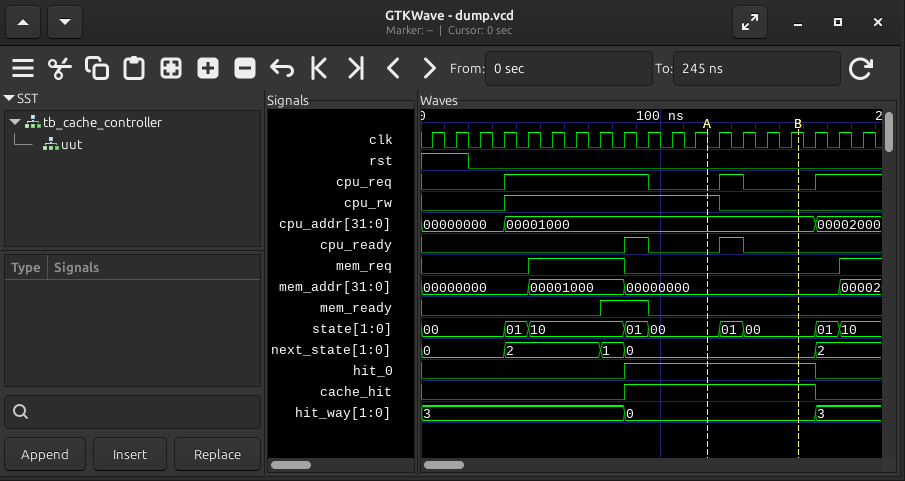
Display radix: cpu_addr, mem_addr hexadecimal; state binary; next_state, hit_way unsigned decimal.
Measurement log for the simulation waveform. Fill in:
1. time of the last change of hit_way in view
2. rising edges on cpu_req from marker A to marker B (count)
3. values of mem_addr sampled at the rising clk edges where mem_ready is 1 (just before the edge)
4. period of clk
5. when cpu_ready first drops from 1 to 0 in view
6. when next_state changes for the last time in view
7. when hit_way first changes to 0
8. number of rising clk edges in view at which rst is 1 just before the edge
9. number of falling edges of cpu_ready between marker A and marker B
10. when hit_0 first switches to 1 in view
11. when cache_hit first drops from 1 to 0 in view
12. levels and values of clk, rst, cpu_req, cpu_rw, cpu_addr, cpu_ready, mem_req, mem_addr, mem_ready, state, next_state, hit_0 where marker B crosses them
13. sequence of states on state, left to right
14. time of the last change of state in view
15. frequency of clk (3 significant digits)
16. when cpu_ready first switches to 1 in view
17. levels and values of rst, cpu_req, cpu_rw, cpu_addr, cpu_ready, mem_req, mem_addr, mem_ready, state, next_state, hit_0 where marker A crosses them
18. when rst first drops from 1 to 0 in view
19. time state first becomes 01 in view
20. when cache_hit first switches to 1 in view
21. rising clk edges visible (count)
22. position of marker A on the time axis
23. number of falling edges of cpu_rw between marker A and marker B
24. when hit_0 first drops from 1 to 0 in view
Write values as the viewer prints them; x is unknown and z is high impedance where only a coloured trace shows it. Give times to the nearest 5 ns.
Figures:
165 ns
1
00001000, 00000000
10 ns
95 ns
165 ns
85 ns
2
1
85 ns
165 ns
clk=1, rst=0, cpu_req=0, cpu_rw=0, cpu_addr=00001000, cpu_ready=0, mem_req=0, mem_addr=00000000, mem_ready=0, state=00, next_state=0, hit_0=1
00, 01, 10, 01, 00, 01, 00, 01, 10
175 ns
100 MHz
85 ns
rst=0, cpu_req=0, cpu_rw=1, cpu_addr=00001000, cpu_ready=0, mem_req=0, mem_addr=00000000, mem_ready=0, state=00, next_state=0, hit_0=1
20 ns
35 ns
85 ns
19
120 ns
1
165 ns
